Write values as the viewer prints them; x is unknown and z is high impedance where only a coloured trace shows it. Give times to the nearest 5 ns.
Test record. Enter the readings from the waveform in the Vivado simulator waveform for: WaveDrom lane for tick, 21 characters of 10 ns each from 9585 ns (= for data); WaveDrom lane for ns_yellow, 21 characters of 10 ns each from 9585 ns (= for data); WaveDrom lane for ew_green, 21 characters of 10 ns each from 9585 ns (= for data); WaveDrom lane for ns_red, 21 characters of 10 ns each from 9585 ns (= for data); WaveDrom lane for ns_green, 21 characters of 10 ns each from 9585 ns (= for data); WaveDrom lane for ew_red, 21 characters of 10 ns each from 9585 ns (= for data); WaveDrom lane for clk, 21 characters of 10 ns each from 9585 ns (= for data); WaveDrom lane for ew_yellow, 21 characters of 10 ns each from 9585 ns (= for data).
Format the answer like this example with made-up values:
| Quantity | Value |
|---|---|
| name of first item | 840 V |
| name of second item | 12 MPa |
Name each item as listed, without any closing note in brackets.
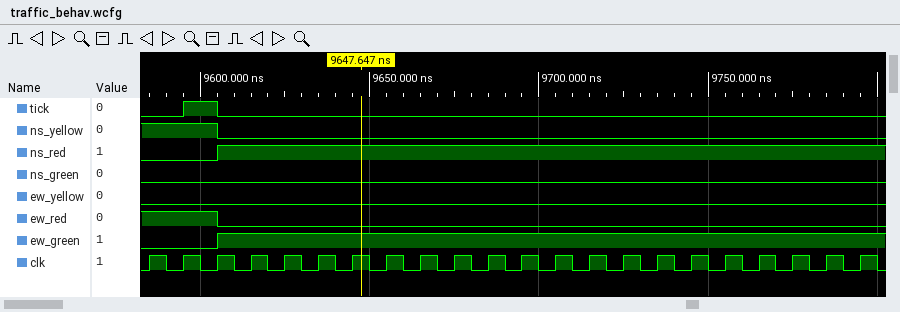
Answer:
| Quantity | Value |
|---|---|
| WaveDrom lane for tick, 21 characters of 10 ns each from 9585 ns | {name: 'tick', wave: '010..................'} |
| WaveDrom lane for ns_yellow, 21 characters of 10 ns each from 9585 ns | {name: 'ns_yellow', wave: '1.0..................'} |
| WaveDrom lane for ew_green, 21 characters of 10 ns each from 9585 ns | {name: 'ew_green', wave: '0.1..................'} |
| WaveDrom lane for ns_red, 21 characters of 10 ns each from 9585 ns | {name: 'ns_red', wave: '0.1..................'} |
| WaveDrom lane for ns_green, 21 characters of 10 ns each from 9585 ns | {name: 'ns_green', wave: '0....................'} |
| WaveDrom lane for ew_red, 21 characters of 10 ns each from 9585 ns | {name: 'ew_red', wave: '1.0..................'} |
| WaveDrom lane for clk, 21 characters of 10 ns each from 9585 ns | {name: 'clk', wave: 'p....................'} |
| WaveDrom lane for ew_yellow, 21 characters of 10 ns each from 9585 ns | {name: 'ew_yellow', wave: '0....................'} |
